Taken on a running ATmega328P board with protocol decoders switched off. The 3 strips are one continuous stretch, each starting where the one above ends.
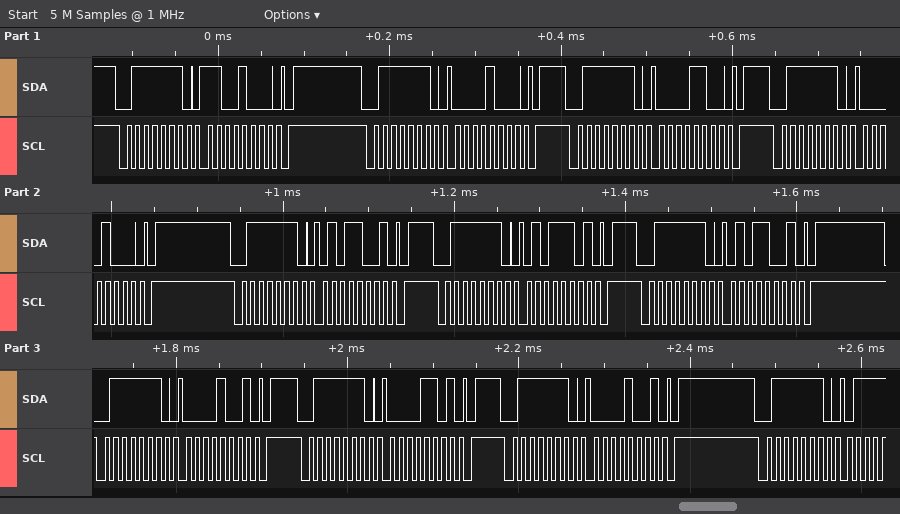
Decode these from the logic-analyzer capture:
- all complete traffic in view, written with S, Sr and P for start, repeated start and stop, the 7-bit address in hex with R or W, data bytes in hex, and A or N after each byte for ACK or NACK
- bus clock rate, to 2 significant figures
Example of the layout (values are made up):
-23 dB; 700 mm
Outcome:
S 3FW A C8 A P S 3FW A 08 A P S 3FW A 0C A P S 3FW A 08 A P S 3FW A 59 A P S 3FW A 5D A P S 3FW A 59 A P S 3FW A 09 A P S 3FW A 0D A P S 3FW A 09 A P S 3FW A; 100 kHz
